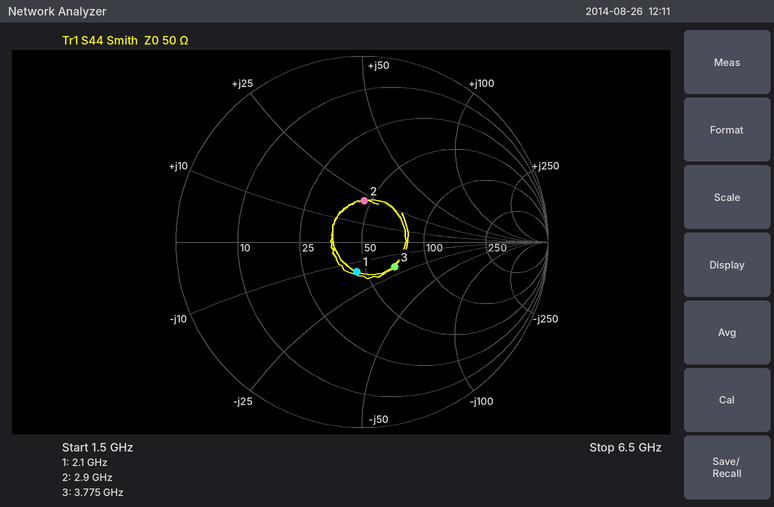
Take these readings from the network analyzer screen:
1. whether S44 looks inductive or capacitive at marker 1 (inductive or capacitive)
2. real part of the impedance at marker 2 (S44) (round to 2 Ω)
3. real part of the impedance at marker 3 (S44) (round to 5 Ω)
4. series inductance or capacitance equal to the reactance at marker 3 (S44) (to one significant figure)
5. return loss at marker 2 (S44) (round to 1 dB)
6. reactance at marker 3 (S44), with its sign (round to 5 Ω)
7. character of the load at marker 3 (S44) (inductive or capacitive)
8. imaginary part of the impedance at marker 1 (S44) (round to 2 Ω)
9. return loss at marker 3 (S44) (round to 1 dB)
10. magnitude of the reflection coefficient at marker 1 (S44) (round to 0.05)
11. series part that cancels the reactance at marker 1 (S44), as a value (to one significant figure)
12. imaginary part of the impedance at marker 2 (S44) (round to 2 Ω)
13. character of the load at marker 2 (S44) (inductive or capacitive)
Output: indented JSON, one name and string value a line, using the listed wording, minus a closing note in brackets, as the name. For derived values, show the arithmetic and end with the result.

{
  "whether S44 looks inductive or capacitive at marker 1": "capacitive",
  "real part of the impedance at marker 2 (S44)": "46 Ω",
  "real part of the impedance at marker 3 (S44)": "70 Ω",
  "series inductance or capacitance equal to the reactance at marker 3 (S44)": "C = 1/(2π × 3.775 GHz × 20 Ω) ≈ 2 pF",
  "return loss at marker 2 (S44)": "13 dB",
  "reactance at marker 3 (S44), with its sign": "-20 Ω",
  "character of the load at marker 3 (S44)": "capacitive",
  "imaginary part of the impedance at marker 1 (S44)": "-14 Ω",
  "return loss at marker 3 (S44)": "13 dB",
  "magnitude of the reflection coefficient at marker 1 (S44)": "0.15",
  "series part that cancels the reactance at marker 1 (S44), as a value": "L = 14 Ω/(2π × 2.1 GHz) ≈ 1 nH",
  "imaginary part of the impedance at marker 2 (S44)": "+22 Ω",
  "character of the load at marker 2 (S44)": "inductive"
}
